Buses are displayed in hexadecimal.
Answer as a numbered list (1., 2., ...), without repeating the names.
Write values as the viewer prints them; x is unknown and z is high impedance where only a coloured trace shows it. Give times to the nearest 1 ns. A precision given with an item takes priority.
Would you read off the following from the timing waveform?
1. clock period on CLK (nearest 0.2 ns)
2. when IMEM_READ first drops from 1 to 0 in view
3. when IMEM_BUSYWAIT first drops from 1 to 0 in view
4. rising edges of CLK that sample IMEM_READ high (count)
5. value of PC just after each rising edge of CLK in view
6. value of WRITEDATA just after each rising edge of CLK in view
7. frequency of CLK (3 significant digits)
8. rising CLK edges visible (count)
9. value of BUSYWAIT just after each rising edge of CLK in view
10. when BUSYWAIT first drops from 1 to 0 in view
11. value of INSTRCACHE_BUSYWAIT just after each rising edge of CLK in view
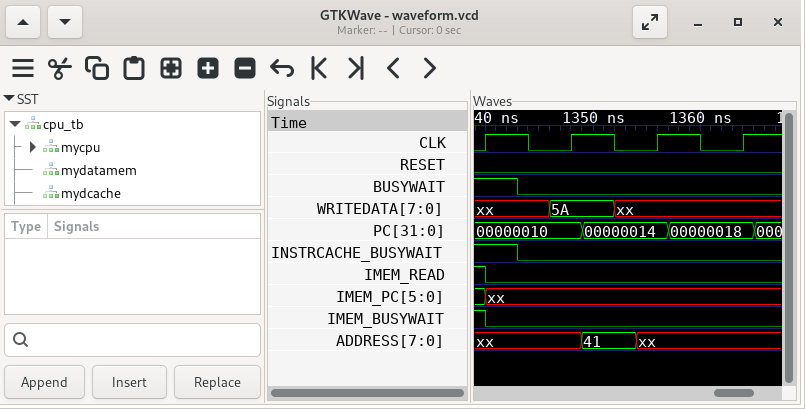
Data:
1. 8 ns
2. 1340 ns
3. 1340 ns
4. 1
5. 00000010, 00000010, 00000014, 00000018
6. xx, 5A, xx, xx
7. 125 MHz
8. 4
9. 1 0 0 0
10. 1343 ns
11. 1 0 0 0
